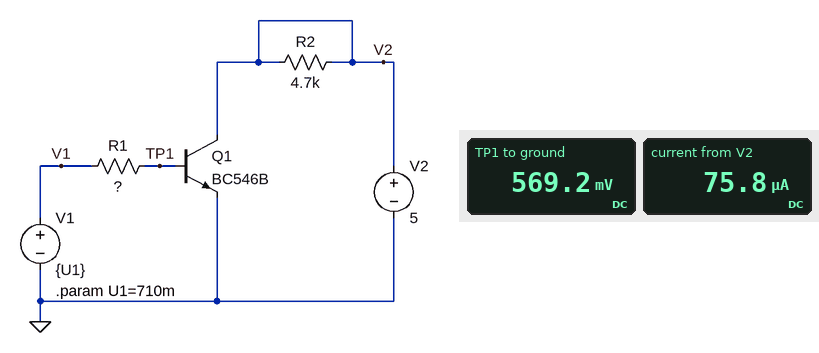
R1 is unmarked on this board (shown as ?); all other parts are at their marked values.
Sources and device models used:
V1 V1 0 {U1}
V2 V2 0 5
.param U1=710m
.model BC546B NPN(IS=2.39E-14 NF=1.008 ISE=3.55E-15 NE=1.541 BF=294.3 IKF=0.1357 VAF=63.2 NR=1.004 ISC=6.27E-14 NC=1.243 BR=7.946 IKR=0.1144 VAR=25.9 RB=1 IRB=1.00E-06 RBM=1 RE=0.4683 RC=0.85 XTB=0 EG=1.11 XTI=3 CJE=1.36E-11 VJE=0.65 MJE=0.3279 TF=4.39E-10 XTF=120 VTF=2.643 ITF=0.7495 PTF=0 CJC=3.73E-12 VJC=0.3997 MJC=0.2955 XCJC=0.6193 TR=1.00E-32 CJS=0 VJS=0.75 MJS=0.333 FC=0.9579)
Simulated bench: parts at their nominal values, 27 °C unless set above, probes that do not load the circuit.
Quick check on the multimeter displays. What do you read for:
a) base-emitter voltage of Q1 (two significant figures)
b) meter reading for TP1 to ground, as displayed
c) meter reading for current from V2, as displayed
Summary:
570 mV
569.2 mV
75.8 µA
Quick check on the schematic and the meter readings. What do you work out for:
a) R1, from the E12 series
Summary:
560 kΩ
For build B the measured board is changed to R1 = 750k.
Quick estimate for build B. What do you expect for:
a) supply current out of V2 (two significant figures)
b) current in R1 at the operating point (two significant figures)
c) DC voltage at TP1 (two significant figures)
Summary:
59 µA
200 nA
560 mV
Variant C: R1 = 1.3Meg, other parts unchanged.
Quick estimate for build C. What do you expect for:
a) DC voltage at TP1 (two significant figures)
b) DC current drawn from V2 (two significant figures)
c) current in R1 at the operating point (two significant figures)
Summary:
550 mV
37 µA
120 nA
